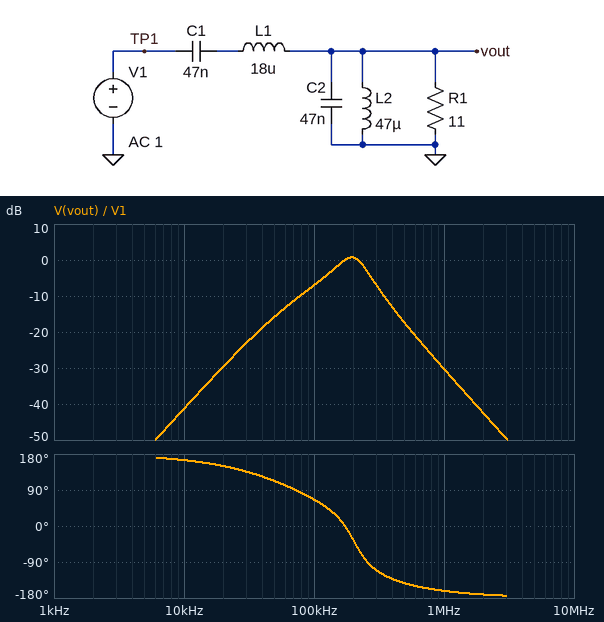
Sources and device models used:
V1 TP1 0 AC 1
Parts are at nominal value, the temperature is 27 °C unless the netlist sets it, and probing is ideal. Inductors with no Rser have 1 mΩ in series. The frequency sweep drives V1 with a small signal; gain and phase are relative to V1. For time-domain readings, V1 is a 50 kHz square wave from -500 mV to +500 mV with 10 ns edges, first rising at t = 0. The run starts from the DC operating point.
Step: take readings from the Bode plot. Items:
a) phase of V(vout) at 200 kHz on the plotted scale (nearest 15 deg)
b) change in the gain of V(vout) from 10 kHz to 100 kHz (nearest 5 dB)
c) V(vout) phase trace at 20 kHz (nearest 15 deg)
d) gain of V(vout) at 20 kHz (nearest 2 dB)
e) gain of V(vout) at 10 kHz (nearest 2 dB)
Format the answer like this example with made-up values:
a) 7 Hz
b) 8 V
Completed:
a) -30 deg
b) 35 dB
c) 150 deg
d) -30 dB
e) -42 dB
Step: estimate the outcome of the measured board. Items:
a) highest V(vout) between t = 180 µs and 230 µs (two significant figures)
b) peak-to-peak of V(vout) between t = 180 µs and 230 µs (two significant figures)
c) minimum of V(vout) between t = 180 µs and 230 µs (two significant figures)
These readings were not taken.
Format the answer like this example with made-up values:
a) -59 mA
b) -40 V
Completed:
a) 340 mV
b) 690 mV
c) -340 mV
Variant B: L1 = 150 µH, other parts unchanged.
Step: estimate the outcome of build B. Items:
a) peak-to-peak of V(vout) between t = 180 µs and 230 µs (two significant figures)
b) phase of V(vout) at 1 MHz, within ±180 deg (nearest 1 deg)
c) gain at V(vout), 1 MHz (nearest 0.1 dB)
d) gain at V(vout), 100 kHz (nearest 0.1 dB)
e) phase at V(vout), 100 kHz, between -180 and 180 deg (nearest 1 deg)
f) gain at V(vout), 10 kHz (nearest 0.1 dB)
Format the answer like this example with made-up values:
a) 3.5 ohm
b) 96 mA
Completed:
a) 650 mV
b) -163 deg
c) -49.1 dB
d) -15.0 dB
e) -77 deg
f) -41.1 dB
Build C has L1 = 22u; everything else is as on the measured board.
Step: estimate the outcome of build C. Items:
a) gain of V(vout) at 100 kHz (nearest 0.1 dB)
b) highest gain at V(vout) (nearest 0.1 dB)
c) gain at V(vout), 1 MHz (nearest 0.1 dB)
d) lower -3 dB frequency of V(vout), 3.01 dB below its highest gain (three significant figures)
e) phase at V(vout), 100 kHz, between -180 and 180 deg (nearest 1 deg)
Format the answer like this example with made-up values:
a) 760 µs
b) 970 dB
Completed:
a) -6.2 dB
b) 0.5 dB
c) -32.1 dB
d) 129 kHz
e) 63 deg
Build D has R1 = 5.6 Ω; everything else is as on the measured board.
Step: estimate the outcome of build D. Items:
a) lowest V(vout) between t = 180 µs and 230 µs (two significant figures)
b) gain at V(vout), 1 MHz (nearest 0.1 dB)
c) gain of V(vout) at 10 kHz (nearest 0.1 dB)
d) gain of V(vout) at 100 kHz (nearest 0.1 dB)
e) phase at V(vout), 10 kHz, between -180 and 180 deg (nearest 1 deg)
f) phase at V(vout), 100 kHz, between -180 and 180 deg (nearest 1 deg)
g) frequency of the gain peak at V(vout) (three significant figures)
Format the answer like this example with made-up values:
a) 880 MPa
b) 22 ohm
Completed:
a) -220 mV
b) -31.3 dB
c) -42.1 dB
d) -12.3 dB
e) 152 deg
f) 77 deg
g) 178 kHz
